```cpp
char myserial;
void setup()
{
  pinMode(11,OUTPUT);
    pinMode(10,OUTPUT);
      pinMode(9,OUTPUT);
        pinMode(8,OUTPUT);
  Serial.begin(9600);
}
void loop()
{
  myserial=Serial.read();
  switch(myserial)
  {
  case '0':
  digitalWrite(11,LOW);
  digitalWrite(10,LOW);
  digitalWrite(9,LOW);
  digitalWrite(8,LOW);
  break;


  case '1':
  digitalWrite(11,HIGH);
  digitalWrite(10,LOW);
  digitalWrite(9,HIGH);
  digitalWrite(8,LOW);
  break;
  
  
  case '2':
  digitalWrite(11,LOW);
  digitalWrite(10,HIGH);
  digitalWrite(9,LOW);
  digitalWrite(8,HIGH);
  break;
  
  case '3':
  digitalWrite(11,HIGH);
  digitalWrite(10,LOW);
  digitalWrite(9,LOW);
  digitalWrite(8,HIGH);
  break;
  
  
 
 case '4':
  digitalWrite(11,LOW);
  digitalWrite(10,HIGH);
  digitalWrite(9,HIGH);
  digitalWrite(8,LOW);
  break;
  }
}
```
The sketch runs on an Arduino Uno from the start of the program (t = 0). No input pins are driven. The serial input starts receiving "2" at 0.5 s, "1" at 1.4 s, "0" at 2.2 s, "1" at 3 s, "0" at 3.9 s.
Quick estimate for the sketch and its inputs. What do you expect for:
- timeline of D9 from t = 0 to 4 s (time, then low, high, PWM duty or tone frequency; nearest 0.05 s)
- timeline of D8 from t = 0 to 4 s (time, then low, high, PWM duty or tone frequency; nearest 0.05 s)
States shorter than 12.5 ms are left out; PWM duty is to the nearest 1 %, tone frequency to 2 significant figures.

0 s low; 1.4 s high; 2.2 s low; 3 s high; 3.9 s low
0 s low; 0.5 s high; 1.4 s low
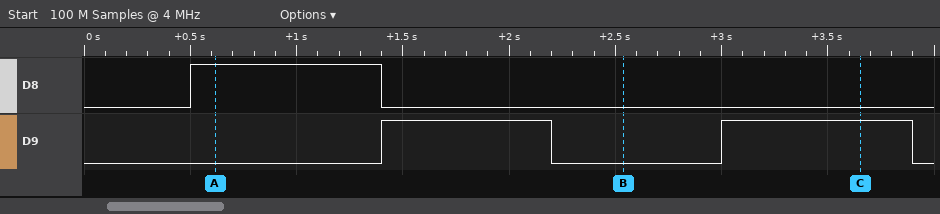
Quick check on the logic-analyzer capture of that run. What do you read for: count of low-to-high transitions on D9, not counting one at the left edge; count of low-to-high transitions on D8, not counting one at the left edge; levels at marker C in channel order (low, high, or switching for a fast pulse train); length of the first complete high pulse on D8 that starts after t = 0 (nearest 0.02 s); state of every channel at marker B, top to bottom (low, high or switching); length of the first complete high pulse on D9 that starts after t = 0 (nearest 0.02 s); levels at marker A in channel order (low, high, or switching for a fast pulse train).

2
1
D8 low, D9 high
0.90 s
D8 low, D9 low
0.80 s
D8 high, D9 low
